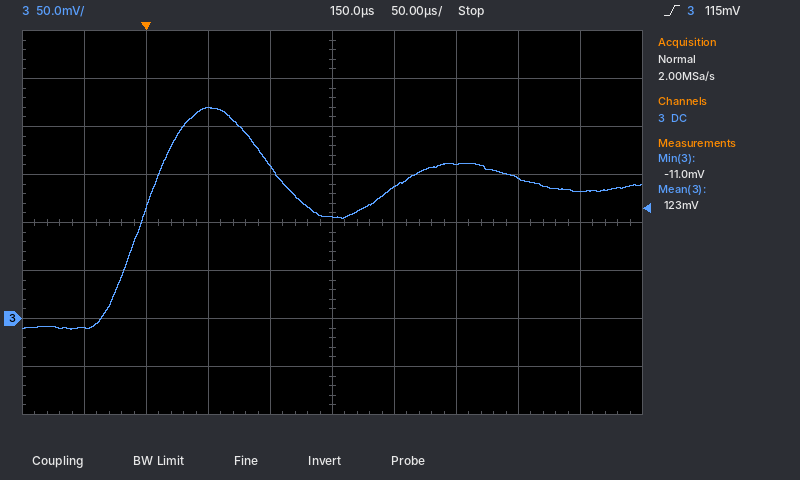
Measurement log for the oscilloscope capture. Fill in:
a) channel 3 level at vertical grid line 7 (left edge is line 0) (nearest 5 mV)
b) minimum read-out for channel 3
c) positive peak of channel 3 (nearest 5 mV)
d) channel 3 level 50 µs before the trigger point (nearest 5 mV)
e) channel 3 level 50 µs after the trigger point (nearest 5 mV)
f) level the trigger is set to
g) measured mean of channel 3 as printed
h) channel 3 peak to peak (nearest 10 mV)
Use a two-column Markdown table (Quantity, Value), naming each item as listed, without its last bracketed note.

| Quantity | Value |
|---|---|
| channel 3 level at vertical grid line 7 (left edge is line 0) | 160 mV |
| minimum read-out for channel 3 | -11.0 mV |
| positive peak of channel 3 | 220 mV |
| channel 3 level 50 µs before the trigger point | -10 mV |
| channel 3 level 50 µs after the trigger point | 220 mV |
| level the trigger is set to | 115 mV |
| measured mean of channel 3 as printed | 123 mV |
| channel 3 peak to peak | 230 mV |
